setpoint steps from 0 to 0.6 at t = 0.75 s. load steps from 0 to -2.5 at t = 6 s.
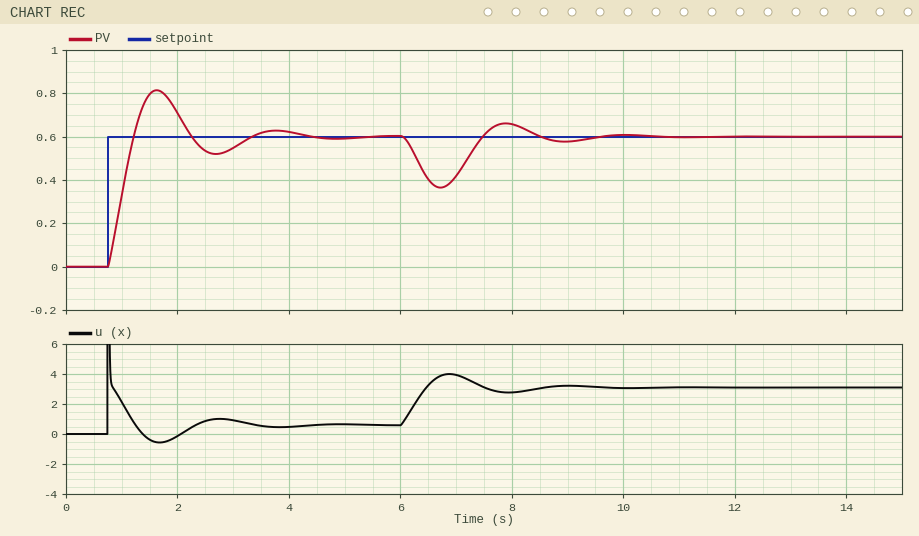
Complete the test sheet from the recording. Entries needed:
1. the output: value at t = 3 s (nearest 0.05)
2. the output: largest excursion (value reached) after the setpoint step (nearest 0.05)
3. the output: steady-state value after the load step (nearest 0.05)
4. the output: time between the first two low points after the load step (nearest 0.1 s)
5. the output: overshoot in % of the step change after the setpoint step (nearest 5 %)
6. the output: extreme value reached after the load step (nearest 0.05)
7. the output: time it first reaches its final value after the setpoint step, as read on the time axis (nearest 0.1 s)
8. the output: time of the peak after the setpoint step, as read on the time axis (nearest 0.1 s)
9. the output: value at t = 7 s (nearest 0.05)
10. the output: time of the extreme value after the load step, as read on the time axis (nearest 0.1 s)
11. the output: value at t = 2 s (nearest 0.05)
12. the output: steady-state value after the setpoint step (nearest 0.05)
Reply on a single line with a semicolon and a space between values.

0.55; 0.80; 0.60; 2.2 s; 35 %; 0.35; 1.2 s; 1.6 s; 0.40; 6.7 s; 0.70; 0.60
